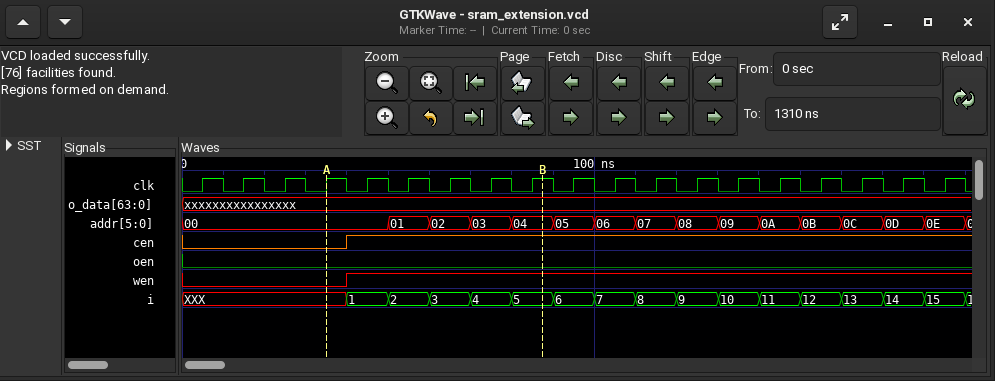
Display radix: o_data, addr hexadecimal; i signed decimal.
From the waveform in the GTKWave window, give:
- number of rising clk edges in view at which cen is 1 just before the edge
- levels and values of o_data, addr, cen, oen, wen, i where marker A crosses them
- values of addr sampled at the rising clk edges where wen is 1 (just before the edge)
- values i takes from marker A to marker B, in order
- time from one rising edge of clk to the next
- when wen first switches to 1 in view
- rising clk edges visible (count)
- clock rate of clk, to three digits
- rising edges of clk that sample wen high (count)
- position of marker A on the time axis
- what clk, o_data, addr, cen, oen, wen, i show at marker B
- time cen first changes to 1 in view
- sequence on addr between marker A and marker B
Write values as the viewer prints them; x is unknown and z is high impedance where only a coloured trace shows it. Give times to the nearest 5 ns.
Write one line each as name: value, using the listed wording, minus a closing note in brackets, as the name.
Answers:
number of rising clk edges in view at which cen is 1 just before the edge: 15
levels and values of o_data, addr, cen, oen, wen, i where marker A crosses them: o_data=xxxxxxxxxxxxxxxx, addr=00, cen=0, oen=0, wen=0, i=XXX
values of addr sampled at the rising clk edges where wen is 1: 00, 01, 02, 03, 04, 05, 06, 07, 08, 09, 0A, 0B, 0C, 0D, 0E
values i takes from marker A to marker B, in order: XXX, 1, 2, 3, 4, 5
time from one rising edge of clk to the next: 10 ns
when wen first switches to 1 in view: 40 ns
rising clk edges visible: 19
clock rate of clk, to three digits: 100 MHz
rising edges of clk that sample wen high: 15
position of marker A on the time axis: 35 ns
what clk, o_data, addr, cen, oen, wen, i show at marker B: clk=1, o_data=xxxxxxxxxxxxxxxx, addr=04, cen=1, oen=0, wen=1, i=5
time cen first changes to 1 in view: 40 ns
sequence on addr between marker A and marker B: 00, 01, 02, 03, 04
